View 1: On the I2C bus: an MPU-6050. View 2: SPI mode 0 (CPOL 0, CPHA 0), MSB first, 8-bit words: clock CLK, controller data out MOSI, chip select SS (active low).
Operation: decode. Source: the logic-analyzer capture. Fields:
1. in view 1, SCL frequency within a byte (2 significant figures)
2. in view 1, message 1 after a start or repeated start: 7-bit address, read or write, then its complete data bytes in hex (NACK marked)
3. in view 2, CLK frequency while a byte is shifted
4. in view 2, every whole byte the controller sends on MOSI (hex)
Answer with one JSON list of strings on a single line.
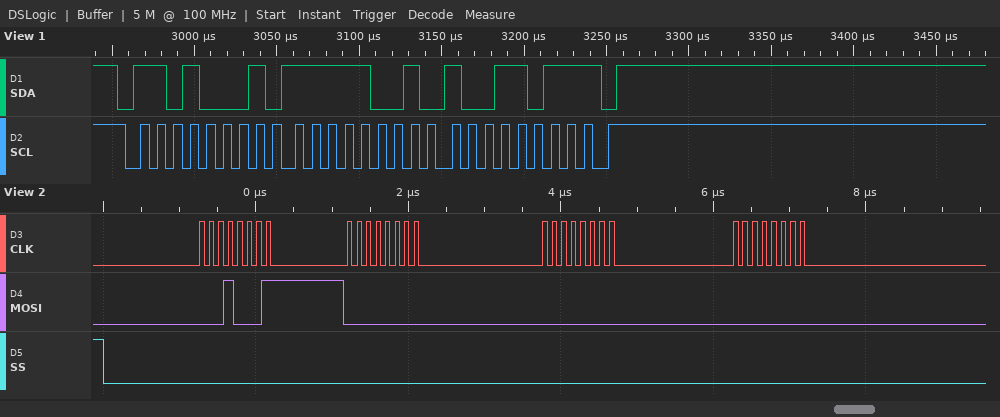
["100 kHz", "0x68 read: F9 9B NACK", "8 MHz", "11 00 00 00"]
